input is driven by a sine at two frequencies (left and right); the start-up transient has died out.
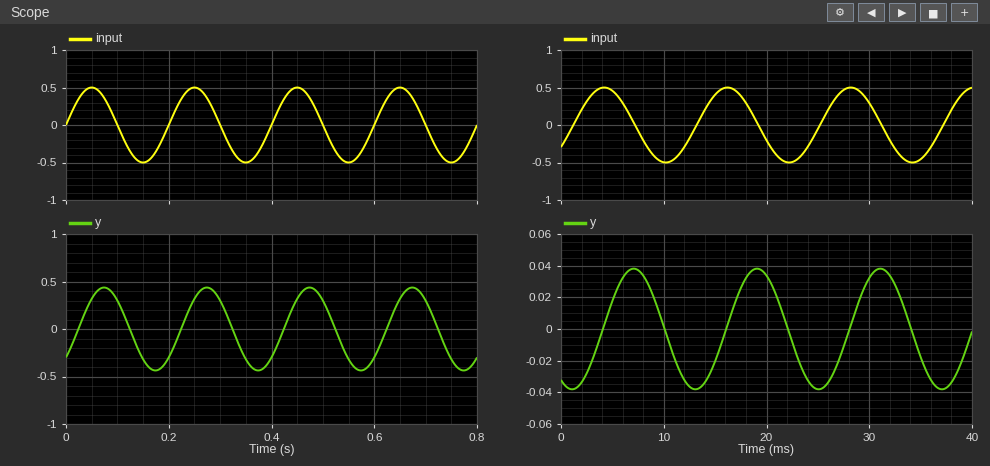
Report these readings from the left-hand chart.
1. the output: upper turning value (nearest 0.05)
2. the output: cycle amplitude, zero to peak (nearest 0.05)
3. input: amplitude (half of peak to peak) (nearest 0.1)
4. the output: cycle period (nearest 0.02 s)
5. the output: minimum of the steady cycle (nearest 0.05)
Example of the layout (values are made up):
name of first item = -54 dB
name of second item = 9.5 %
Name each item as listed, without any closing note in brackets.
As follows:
the output: upper turning value = 0.45
the output: cycle amplitude, zero to peak = 0.45
input: amplitude (half of peak to peak) = 0.5
the output: cycle period = 0.20 s
the output: minimum of the steady cycle = -0.45
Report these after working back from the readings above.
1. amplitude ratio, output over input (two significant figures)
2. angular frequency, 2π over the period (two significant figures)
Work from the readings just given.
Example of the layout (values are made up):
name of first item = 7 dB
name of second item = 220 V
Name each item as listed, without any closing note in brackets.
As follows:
amplitude ratio, output over input = 0.90
angular frequency, 2π over the period = 31 rad/s
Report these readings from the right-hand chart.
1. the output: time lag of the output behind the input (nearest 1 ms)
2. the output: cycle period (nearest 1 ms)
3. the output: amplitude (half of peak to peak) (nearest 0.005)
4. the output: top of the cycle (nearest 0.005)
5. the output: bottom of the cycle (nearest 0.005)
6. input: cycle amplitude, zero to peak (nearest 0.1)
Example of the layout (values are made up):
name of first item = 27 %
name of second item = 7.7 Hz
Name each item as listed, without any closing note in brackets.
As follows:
the output: time lag of the output behind the input = 3 ms
the output: cycle period = 12 ms
the output: amplitude (half of peak to peak) = 0.040
the output: top of the cycle = 0.040
the output: bottom of the cycle = -0.040
input: cycle amplitude, zero to peak = 0.5
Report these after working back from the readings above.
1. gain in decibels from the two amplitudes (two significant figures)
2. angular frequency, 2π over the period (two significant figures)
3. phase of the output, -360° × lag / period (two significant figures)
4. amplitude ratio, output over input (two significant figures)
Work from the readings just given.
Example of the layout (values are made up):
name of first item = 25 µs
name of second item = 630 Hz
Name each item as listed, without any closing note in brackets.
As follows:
gain in decibels from the two amplitudes = -22 dB
angular frequency, 2π over the period = 0.52 rad/ms
phase of the output, -360° × lag / period = -90°
amplitude ratio, output over input = 0.080
